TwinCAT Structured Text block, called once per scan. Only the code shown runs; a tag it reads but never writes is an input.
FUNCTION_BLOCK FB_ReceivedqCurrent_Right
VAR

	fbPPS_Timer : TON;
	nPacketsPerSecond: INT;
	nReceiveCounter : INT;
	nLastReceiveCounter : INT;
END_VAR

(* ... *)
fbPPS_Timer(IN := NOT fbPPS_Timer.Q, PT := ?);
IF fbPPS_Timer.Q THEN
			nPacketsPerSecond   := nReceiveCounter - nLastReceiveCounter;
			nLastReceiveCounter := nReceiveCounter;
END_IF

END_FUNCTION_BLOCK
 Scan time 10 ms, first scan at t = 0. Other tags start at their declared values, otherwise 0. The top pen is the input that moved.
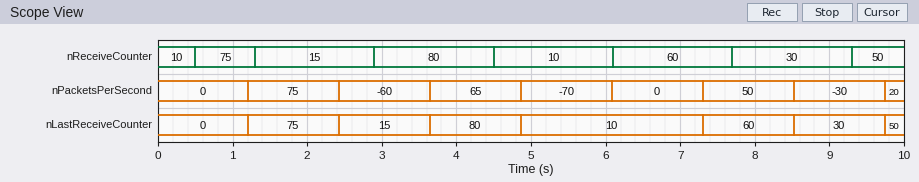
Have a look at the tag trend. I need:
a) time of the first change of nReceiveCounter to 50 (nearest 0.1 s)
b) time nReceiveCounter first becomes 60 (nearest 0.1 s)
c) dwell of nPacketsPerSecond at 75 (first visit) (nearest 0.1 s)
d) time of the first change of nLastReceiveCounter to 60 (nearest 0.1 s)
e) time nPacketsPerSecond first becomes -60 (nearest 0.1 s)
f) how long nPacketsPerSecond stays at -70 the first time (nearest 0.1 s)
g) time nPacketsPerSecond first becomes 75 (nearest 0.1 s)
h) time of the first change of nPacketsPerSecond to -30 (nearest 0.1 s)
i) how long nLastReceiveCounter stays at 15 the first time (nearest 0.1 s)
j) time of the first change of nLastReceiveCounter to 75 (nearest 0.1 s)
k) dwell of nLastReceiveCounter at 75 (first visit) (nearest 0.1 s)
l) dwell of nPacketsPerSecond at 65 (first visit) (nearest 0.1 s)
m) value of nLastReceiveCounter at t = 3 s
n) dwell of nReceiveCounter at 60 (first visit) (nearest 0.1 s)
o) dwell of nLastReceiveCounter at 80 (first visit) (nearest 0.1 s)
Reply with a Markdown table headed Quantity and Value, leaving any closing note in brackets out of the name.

| Quantity | Value |
|---|---|
| time of the first change of nReceiveCounter to 50 | 9.3 s |
| time nReceiveCounter first becomes 60 | 6.1 s |
| dwell of nPacketsPerSecond at 75 (first visit) | 1.2 s |
| time of the first change of nLastReceiveCounter to 60 | 7.3 s |
| time nPacketsPerSecond first becomes -60 | 2.4 s |
| how long nPacketsPerSecond stays at -70 the first time | 1.2 s |
| time nPacketsPerSecond first becomes 75 | 1.2 s |
| time of the first change of nPacketsPerSecond to -30 | 8.5 s |
| how long nLastReceiveCounter stays at 15 the first time | 1.2 s |
| time of the first change of nLastReceiveCounter to 75 | 1.2 s |
| dwell of nLastReceiveCounter at 75 (first visit) | 1.2 s |
| dwell of nPacketsPerSecond at 65 (first visit) | 1.2 s |
| value of nLastReceiveCounter at t = 3 s | 15 |
| dwell of nReceiveCounter at 60 (first visit) | 1.6 s |
| dwell of nLastReceiveCounter at 80 (first visit) | 1.2 s |
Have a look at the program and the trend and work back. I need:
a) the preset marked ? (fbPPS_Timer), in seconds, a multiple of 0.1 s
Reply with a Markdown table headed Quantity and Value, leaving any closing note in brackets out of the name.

| Quantity | Value |
|---|---|
| the preset marked ? (fbPPS_Timer), in seconds, a multiple of 0.1 s | 1.2 s |
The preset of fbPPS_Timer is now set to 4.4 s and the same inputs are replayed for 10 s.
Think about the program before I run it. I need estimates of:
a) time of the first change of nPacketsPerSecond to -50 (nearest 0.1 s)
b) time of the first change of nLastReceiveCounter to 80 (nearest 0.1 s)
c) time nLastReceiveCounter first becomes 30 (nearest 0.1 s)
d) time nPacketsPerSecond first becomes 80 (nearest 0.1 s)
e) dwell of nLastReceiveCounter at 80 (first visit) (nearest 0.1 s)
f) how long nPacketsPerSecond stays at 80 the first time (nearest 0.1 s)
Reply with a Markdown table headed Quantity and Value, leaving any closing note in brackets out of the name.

| Quantity | Value |
|---|---|
| time of the first change of nPacketsPerSecond to -50 | 8.8 s |
| time of the first change of nLastReceiveCounter to 80 | 4.4 s |
| time nLastReceiveCounter first becomes 30 | 8.8 s |
| time nPacketsPerSecond first becomes 80 | 4.4 s |
| dwell of nLastReceiveCounter at 80 (first visit) | 4.4 s |
| how long nPacketsPerSecond stays at 80 the first time | 4.4 s |
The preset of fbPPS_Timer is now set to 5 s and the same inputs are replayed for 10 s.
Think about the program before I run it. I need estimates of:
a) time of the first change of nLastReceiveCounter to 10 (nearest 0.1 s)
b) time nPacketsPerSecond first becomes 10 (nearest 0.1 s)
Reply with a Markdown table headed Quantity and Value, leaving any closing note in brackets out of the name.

| Quantity | Value |
|---|---|
| time of the first change of nLastReceiveCounter to 10 | 5.0 s |
| time nPacketsPerSecond first becomes 10 | 5.0 s |
